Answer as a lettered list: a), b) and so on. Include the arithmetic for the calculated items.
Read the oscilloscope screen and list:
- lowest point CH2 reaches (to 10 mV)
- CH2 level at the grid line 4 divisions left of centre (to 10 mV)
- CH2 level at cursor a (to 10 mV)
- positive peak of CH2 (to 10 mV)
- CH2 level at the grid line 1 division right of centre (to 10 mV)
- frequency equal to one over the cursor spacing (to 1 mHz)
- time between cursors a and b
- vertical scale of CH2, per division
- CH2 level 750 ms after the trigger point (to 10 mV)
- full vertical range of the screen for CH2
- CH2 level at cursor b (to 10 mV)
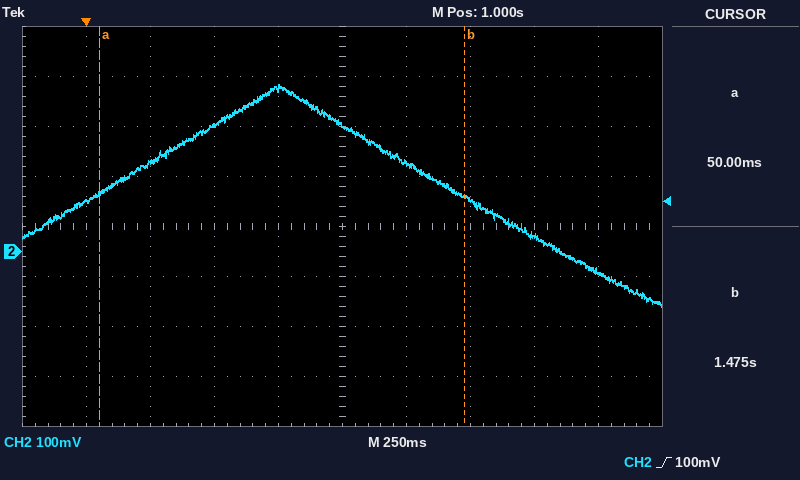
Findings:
a) -110 mV
b) 100 mV
c) 120 mV
d) 330 mV
e) 180 mV
f) 1 / 1.425 s ≈ 702 mHz
g) 1.475 s − (50 ms) = 1.425 s
h) 100 mV
i) 330 mV
j) 800 mV
k) 110 mV
